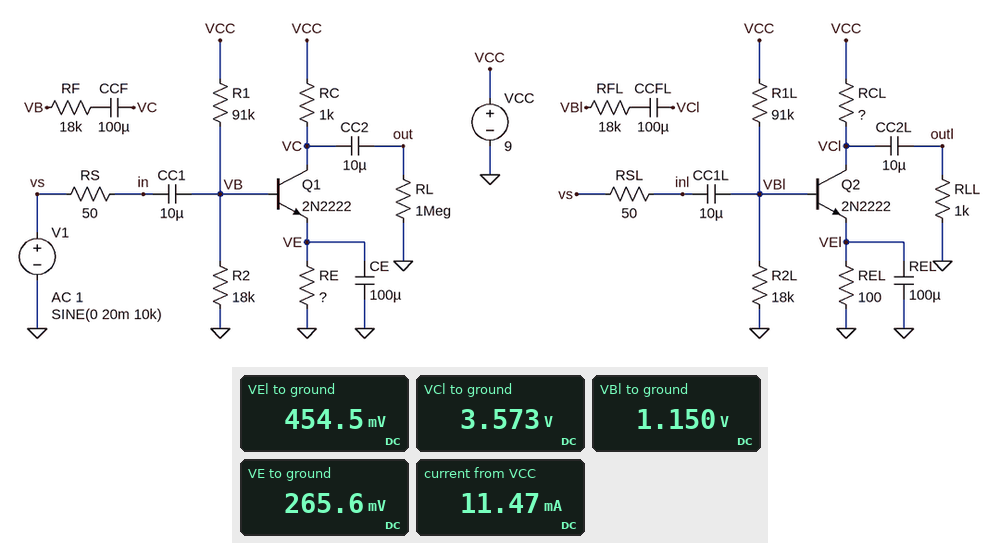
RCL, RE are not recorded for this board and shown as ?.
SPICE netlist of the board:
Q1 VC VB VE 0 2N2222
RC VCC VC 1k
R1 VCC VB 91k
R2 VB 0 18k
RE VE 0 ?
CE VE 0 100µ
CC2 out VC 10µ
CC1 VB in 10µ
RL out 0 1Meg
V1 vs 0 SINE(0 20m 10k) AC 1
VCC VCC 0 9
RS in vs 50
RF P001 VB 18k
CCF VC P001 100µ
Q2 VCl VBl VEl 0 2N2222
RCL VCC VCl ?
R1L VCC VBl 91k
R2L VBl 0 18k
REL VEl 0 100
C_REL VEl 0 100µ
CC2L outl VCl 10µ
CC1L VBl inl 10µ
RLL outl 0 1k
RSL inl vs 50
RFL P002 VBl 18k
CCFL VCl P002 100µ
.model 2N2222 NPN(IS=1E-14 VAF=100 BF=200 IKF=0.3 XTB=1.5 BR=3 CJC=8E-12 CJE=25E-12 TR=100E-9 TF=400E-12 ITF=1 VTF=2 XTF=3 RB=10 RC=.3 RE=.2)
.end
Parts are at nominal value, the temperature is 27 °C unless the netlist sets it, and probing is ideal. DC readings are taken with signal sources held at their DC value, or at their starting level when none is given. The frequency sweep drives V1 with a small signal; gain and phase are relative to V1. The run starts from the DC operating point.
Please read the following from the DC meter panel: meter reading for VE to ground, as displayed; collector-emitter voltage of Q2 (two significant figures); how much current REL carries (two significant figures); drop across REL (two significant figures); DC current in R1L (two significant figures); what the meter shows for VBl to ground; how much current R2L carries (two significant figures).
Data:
265.6 mV
3.1 V
4.5 mA
450 mV
86 µA
1.150 V
64 µA
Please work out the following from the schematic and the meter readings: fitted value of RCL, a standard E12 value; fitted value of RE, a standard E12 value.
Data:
1.2 kΩ
39 Ω
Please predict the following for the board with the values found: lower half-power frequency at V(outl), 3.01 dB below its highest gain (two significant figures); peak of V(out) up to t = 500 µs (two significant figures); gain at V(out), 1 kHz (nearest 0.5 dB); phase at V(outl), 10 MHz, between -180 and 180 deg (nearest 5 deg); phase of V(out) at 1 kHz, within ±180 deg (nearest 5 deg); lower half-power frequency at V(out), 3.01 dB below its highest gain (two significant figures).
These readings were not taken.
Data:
280 Hz
2.4 V
41.5 dB
120 deg
-160 deg
370 Hz
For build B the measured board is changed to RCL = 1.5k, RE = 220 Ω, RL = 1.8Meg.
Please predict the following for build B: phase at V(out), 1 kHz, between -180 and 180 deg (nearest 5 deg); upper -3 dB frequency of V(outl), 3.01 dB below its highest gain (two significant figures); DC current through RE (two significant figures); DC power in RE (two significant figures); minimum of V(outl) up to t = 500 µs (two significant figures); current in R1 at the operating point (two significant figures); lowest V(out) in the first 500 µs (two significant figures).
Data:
-170 deg
4.9 MHz
2.8 mA
1.7 mW
-1.6 V
85 µA
-1.7 V
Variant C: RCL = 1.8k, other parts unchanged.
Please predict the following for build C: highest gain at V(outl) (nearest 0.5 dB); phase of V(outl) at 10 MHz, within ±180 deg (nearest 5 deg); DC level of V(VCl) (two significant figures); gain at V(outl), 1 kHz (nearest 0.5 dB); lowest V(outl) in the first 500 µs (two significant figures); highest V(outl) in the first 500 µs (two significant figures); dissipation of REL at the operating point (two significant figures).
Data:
37.5 dB
105 deg
950 mV
37.0 dB
-450 mV
1.2 V
2.0 mW
